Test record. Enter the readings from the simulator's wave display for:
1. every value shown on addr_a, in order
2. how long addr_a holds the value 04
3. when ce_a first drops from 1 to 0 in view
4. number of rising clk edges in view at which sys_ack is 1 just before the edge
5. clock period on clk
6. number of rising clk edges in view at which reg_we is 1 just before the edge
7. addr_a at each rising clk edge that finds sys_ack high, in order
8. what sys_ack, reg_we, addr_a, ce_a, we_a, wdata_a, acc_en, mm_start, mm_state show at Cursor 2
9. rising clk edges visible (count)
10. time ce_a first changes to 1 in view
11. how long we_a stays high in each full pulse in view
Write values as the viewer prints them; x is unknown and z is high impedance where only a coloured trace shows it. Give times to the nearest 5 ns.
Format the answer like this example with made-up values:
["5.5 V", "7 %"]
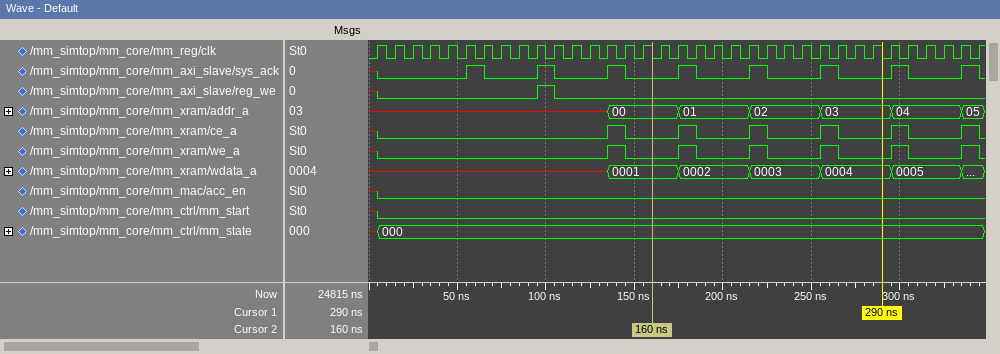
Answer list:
["x, 00, 01, 02, 03, 04, 05", "40 ns", "145 ns", "8", "10 ns", "1", "x, x, 00, 01, 02, 03, 04, 05", "sys_ack=0, reg_we=0, addr_a=00, ce_a=0, we_a=0, wdata_a=0001, acc_en=0, mm_start=0, mm_state=000", "35", "135 ns", "10 ns, 10 ns, 10 ns, 10 ns, 10 ns, 10 ns"]
